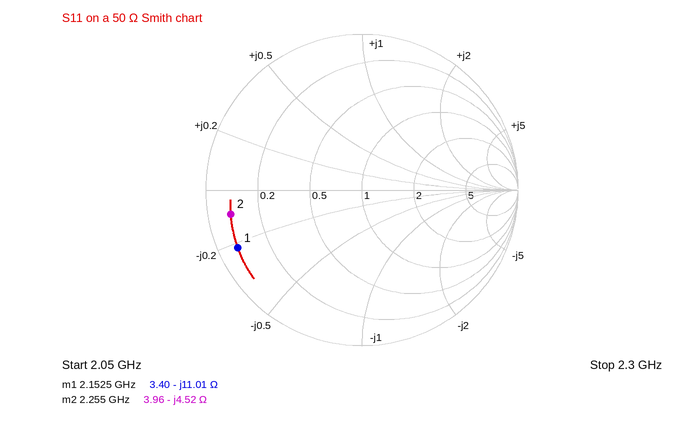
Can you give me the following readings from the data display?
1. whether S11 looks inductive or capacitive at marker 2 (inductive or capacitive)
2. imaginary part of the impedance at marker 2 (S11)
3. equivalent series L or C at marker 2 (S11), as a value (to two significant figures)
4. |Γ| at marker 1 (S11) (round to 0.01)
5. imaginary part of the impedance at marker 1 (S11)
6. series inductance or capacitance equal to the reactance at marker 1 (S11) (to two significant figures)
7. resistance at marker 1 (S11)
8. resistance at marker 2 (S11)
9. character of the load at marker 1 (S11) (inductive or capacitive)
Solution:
capacitive
-4.52 Ω
16 pF
0.88
-11.01 Ω
6.7 pF
3.40 Ω
3.96 Ω
capacitive
